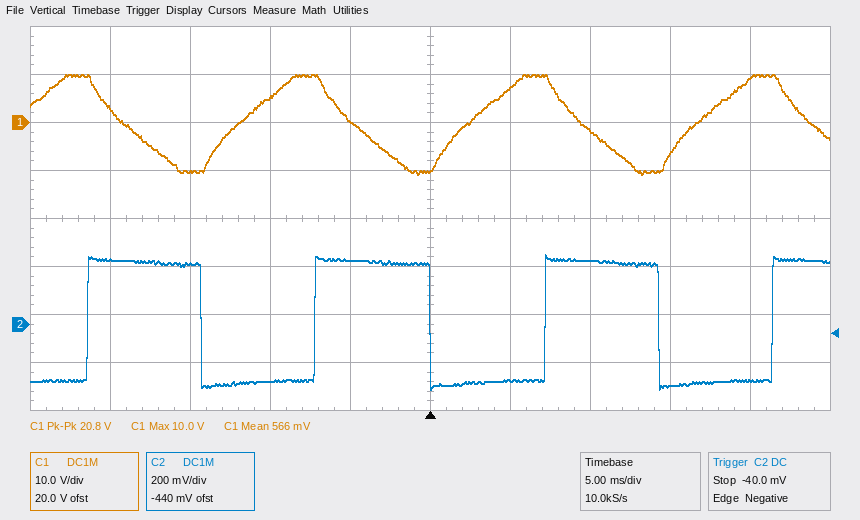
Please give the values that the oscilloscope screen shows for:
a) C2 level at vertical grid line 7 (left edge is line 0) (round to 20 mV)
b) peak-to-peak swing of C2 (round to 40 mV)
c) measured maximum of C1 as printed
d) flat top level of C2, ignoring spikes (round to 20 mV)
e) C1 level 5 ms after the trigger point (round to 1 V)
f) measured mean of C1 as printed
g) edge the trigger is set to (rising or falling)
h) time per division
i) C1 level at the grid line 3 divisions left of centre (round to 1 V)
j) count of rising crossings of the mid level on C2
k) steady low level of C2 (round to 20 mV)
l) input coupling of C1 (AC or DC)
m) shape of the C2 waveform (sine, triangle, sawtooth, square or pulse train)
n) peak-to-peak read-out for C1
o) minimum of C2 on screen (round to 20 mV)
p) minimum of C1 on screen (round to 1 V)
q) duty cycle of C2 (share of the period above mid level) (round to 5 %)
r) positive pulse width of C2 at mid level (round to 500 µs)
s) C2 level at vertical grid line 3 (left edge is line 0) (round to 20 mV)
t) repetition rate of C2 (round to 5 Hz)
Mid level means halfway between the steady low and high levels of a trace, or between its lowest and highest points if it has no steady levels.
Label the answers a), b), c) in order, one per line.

a) 260 mV
b) 560 mV
c) 10.0 V
d) 260 mV
e) 7 V
f) 566 mV
g) falling
h) 5 ms
i) -10 V
j) 4
k) -240 mV
l) DC
m) square
n) 20.8 V
o) -280 mV
p) -11 V
q) 50 %
r) 7.0 ms
s) -240 mV
t) 70 Hz
